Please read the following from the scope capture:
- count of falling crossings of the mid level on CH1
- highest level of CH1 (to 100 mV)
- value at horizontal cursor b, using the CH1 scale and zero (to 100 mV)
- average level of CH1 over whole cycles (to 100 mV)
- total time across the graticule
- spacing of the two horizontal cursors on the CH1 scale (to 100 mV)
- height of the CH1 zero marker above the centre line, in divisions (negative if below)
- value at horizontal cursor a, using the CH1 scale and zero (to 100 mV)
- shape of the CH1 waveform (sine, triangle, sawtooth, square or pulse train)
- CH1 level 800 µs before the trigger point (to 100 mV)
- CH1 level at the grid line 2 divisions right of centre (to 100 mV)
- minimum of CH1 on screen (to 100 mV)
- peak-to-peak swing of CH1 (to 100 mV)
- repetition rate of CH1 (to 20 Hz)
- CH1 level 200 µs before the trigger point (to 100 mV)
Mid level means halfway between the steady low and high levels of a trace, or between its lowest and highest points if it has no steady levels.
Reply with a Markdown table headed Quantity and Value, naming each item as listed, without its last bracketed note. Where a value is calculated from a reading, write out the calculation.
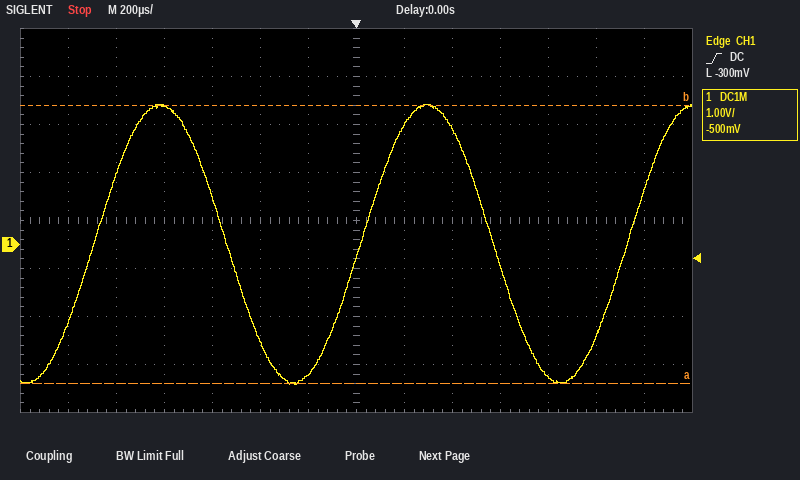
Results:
| Quantity | Value |
|---|---|
| count of falling crossings of the mid level on CH1 | 2 |
| highest level of CH1 | 2.9 V |
| value at horizontal cursor b, using the CH1 scale and zero | 2.9 V |
| average level of CH1 over whole cycles | (2.9 V + (-2.9 V)) / 2 ≈ 0.0 V |
| total time across the graticule | 2.8 ms |
| spacing of the two horizontal cursors on the CH1 scale | 5.8 V |
| height of the CH1 zero marker above the centre line, in divisions | -0.5 div |
| value at horizontal cursor a, using the CH1 scale and zero | -2.9 V |
| shape of the CH1 waveform | sine |
| CH1 level 800 µs before the trigger point | 2.9 V |
| CH1 level at the grid line 2 divisions right of centre | 2.4 V |
| minimum of CH1 on screen | -2.9 V |
| peak-to-peak swing of CH1 | 2.9 V − (-2.9 V) = 5.8 V |
| repetition rate of CH1 | 900 Hz |
| CH1 level 200 µs before the trigger point | -2.7 V |
